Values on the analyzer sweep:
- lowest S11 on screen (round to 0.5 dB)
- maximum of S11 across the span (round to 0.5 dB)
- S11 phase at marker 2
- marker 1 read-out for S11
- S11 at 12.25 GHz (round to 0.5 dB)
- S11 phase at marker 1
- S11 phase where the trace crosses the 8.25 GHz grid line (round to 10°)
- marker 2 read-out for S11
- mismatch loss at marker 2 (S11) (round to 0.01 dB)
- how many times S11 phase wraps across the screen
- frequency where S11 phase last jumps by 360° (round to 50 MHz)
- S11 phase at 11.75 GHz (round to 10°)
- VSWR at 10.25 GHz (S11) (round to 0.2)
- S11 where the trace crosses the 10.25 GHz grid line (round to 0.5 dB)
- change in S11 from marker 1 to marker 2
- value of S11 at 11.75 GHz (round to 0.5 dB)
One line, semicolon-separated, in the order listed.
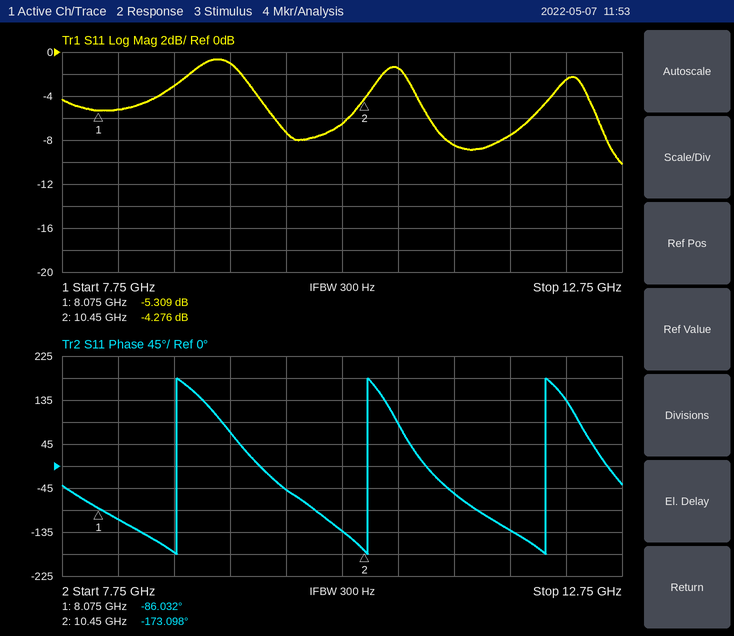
-10.0 dB; -0.5 dB; -173.098°; -5.309 dB; -2.5 dB; -86.032°; -110°; -4.276 dB; 2.03 dB; 3; 12.05 GHz; -130°; 2.8; -6.5 dB; 1.033 dB; -7.5 dB
